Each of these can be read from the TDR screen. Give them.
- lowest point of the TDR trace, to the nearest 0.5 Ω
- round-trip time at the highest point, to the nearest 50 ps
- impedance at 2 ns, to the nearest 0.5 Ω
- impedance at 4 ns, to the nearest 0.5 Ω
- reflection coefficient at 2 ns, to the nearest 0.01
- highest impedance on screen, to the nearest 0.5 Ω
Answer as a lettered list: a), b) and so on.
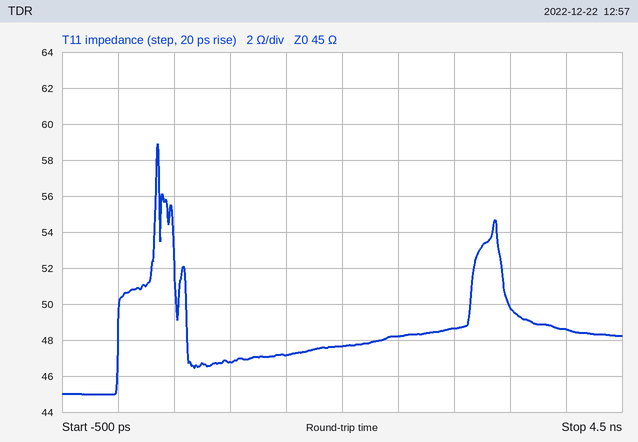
a) 45.0 Ω
b) 350 ps
c) 47.5 Ω
d) 48.5 Ω
e) +0.03
f) 59.0 Ω
